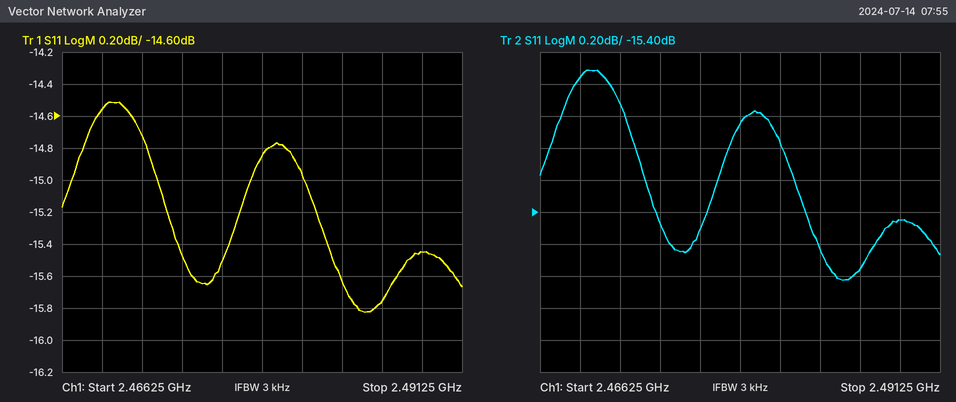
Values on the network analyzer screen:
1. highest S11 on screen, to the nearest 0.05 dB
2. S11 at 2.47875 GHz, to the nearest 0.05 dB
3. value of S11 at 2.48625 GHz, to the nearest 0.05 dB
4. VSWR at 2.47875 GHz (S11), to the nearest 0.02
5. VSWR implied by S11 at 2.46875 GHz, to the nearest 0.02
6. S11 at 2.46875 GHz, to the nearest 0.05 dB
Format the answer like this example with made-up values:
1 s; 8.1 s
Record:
-14.50 dB; -14.85 dB; -15.75 dB; 1.44; 1.46; -14.55 dB
